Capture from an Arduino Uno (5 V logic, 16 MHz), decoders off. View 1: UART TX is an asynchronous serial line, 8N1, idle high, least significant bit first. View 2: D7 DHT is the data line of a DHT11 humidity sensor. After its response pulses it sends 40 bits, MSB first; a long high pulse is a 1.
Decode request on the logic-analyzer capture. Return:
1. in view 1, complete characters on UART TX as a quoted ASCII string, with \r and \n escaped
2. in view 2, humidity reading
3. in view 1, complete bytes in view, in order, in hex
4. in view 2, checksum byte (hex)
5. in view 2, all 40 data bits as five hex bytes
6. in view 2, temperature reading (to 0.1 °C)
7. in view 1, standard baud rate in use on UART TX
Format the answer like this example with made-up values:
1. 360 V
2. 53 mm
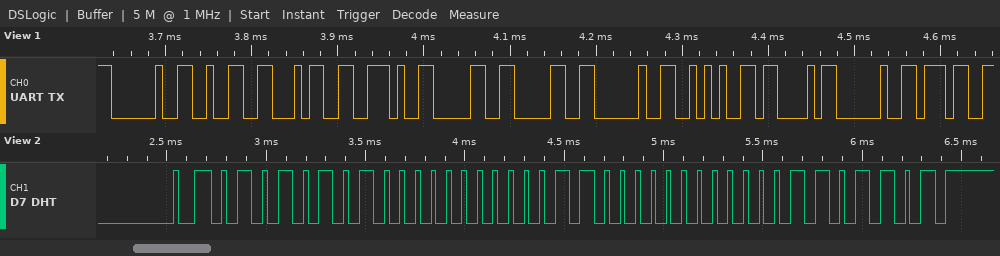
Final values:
1. " 24.00 *C 7"
2. 85 %
3. 20 32 34 2E 30 30 20 2A 43 20 37
4. 0x6D
5. 55 00 18 00 6D
6. 24.0 °C
7. 115200 baud
